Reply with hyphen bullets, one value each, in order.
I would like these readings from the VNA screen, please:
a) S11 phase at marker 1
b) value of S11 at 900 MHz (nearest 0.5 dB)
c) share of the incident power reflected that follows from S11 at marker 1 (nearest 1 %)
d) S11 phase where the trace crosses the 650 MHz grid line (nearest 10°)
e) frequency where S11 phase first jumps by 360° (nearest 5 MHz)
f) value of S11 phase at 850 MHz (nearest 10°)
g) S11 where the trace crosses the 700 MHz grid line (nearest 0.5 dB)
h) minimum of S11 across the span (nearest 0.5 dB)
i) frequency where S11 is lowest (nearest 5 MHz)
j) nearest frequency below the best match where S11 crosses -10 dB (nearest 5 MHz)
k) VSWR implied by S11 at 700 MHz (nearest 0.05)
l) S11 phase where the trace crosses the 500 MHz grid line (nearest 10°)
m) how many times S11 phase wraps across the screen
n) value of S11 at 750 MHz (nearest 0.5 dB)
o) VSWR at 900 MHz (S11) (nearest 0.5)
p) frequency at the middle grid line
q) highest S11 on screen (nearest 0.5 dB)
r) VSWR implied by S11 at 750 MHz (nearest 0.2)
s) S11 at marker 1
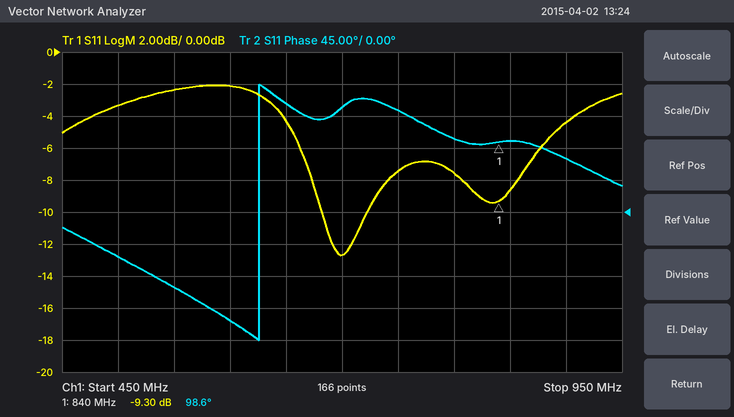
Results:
- 98.6°
- -4.5 dB
- 12 %
- 150°
- 625 MHz
- 100°
- -12.5 dB
- -12.5 dB
- 700 MHz
- 680 MHz
- 1.60
- -60°
- 1
- -7.5 dB
- 4.0
- 700 MHz
- -2.0 dB
- 2.4
- -9.30 dB
